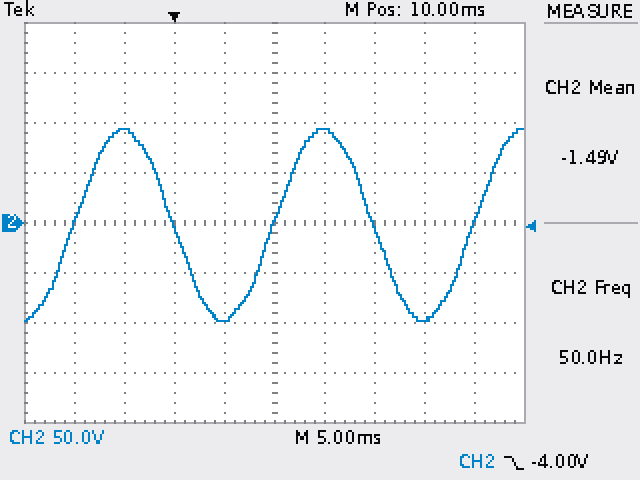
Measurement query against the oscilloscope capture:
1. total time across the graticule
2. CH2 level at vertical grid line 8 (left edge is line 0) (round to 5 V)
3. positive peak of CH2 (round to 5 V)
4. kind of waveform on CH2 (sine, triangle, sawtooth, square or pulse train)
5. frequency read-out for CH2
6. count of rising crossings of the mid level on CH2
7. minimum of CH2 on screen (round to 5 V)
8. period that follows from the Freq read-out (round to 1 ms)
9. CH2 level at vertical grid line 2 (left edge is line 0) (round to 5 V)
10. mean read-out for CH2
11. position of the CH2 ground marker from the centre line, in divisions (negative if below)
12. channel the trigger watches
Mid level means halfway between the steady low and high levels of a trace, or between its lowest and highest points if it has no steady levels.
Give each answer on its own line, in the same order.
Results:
50 ms
-95 V
95 V
sine
50.0 Hz
3
-100 V
20 ms
95 V
-1.49 V
0.0 div
CH2
